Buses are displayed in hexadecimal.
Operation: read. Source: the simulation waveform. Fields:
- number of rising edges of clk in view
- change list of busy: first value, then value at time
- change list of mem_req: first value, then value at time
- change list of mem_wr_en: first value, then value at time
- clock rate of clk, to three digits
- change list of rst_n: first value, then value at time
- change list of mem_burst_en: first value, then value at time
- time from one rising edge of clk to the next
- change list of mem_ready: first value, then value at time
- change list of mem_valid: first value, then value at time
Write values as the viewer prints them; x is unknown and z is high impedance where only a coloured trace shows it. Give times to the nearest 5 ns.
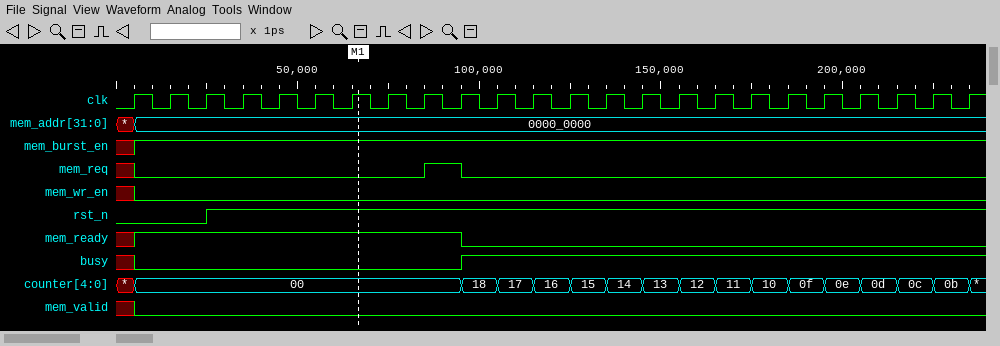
24
x, 0 at 5 ns, 1 at 95 ns
x, 0 at 5 ns, 1 at 85 ns, 0 at 95 ns
x, 0 at 5 ns
100 MHz
0, 1 at 25 ns
x, 1 at 5 ns
10 ns
x, 1 at 5 ns, 0 at 95 ns
x, 0 at 5 ns
